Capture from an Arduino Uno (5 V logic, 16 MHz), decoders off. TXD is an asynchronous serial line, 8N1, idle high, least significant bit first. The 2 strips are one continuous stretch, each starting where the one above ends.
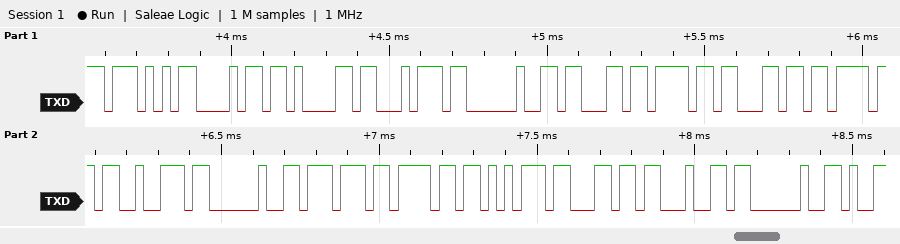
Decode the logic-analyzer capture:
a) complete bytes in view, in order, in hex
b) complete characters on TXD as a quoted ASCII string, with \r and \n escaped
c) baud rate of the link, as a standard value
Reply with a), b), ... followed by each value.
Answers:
a) 0x57 0x68 0x61 0x74 0x20 0x63 0x6F 0x6C 0x6F 0x72 0x20 0x77 0x6F 0x75 0x6C 0x64 0x20
b) "What color would "
c) 38400 baud
